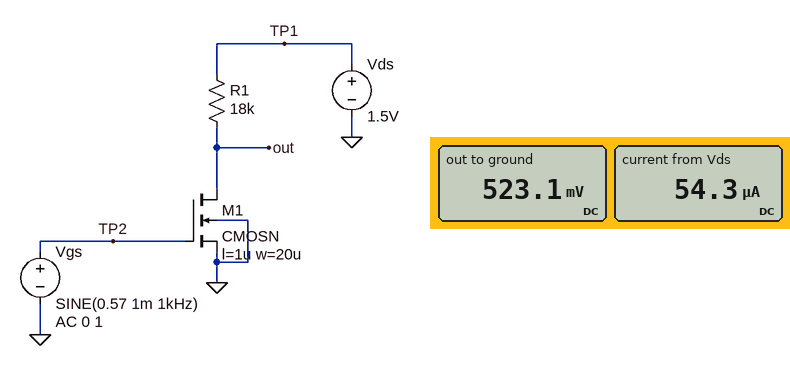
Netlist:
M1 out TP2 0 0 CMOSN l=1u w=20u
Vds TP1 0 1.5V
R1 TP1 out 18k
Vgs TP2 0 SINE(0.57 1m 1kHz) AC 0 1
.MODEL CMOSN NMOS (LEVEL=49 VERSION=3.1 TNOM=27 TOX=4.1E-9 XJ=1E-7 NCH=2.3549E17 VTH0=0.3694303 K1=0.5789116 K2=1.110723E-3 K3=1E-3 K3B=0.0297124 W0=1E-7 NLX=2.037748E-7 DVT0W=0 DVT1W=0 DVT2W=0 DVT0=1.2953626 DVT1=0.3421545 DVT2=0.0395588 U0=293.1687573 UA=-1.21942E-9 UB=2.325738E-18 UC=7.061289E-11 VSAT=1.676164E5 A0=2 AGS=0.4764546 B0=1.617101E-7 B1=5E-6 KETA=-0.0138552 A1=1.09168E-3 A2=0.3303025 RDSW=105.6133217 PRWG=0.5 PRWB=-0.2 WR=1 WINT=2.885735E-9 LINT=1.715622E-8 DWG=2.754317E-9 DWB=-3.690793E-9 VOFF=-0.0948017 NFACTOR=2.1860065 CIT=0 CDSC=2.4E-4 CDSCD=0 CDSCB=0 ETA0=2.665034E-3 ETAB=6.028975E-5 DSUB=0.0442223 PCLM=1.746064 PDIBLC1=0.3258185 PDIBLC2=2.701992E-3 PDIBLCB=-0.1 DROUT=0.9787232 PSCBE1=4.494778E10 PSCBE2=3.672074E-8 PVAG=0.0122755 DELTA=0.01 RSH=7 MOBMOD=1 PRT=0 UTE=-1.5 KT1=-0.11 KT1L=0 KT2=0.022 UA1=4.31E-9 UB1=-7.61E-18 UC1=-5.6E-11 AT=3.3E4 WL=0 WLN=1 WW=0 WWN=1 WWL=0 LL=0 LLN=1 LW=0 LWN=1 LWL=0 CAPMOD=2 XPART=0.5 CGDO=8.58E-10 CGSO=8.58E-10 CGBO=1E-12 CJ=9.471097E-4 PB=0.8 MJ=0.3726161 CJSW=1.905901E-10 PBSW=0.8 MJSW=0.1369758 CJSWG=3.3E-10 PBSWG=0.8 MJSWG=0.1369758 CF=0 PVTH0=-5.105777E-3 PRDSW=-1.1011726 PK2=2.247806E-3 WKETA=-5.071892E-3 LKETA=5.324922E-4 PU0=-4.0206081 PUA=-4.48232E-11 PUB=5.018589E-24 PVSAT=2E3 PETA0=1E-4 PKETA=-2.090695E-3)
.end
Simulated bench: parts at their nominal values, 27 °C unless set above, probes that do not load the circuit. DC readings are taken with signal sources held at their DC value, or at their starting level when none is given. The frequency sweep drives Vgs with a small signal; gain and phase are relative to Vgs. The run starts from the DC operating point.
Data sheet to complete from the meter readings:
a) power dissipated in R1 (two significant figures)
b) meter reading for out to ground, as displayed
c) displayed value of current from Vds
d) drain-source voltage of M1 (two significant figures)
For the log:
53 µW
523.1 mV
54.3 µA
520 mV
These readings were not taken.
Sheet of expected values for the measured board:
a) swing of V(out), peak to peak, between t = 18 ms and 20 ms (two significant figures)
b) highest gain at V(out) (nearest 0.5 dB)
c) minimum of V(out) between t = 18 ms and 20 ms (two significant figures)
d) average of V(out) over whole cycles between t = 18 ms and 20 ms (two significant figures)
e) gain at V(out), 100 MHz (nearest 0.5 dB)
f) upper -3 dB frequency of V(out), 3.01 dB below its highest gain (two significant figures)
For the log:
23 mV
21.0 dB
510 mV
520 mV
21.0 dB
440 MHz
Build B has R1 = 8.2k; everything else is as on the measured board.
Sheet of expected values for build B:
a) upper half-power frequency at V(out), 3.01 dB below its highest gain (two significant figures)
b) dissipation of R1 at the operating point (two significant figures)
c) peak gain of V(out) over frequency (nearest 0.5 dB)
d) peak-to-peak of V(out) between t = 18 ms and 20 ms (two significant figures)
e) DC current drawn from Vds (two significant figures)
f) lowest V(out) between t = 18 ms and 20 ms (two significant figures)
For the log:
1.4 GHz
26 µW
15.0 dB
11 mV
56 µA
1.0 V
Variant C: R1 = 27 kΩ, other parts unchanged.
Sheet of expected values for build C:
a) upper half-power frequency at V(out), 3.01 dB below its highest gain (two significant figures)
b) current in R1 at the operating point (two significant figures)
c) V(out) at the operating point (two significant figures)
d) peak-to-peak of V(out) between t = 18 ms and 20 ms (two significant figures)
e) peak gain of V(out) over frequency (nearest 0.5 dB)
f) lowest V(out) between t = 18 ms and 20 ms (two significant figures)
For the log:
630 MHz
50 µA
150 mV
14 mV
16.5 dB
140 mV
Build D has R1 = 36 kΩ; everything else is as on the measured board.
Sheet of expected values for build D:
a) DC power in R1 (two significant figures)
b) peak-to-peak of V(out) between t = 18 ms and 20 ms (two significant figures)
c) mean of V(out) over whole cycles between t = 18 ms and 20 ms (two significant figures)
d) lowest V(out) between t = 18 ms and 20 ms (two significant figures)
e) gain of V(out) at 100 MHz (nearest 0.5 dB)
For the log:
56 µW
2.6 mV
77 mV
76 mV
2.0 dB
